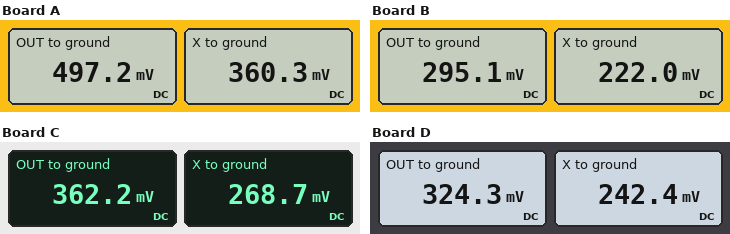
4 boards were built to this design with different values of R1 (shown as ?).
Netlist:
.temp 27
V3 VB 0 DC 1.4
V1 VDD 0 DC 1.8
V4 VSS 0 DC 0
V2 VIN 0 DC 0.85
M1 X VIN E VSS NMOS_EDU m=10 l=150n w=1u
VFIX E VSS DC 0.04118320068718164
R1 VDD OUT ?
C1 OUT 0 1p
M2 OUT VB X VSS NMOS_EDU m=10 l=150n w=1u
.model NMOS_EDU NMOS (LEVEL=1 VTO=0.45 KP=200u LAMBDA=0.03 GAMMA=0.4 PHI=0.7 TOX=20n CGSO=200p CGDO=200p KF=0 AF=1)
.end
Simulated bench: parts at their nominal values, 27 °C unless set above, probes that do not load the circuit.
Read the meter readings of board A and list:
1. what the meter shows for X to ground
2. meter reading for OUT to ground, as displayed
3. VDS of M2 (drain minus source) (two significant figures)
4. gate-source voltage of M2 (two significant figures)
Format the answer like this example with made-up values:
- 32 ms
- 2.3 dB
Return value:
- 360.3 mV
- 497.2 mV
- 140 mV
- 1.0 V
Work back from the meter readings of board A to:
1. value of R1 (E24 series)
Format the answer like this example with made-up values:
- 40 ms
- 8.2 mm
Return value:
- 1.6 kΩ
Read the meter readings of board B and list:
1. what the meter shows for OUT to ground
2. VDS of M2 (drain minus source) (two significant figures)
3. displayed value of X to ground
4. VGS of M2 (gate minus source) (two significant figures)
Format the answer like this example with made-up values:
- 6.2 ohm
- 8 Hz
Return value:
- 295.1 mV
- 73 mV
- 222.0 mV
- 1.2 V
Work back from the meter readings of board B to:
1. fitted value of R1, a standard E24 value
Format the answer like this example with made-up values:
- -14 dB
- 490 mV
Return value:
- 2.4 kΩ
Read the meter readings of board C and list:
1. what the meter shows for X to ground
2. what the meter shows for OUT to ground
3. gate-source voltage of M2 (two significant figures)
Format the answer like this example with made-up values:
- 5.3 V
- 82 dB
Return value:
- 268.7 mV
- 362.2 mV
- 1.1 V
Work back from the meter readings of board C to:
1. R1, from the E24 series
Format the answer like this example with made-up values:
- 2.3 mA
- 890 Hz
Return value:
- 2 kΩ
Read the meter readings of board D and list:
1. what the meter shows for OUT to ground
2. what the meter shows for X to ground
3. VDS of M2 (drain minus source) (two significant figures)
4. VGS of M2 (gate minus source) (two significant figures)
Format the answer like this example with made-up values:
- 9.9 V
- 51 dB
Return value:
- 324.3 mV
- 242.4 mV
- 82 mV
- 1.2 V
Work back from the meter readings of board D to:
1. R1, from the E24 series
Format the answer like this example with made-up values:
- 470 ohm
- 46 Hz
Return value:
- 2.2 kΩ
